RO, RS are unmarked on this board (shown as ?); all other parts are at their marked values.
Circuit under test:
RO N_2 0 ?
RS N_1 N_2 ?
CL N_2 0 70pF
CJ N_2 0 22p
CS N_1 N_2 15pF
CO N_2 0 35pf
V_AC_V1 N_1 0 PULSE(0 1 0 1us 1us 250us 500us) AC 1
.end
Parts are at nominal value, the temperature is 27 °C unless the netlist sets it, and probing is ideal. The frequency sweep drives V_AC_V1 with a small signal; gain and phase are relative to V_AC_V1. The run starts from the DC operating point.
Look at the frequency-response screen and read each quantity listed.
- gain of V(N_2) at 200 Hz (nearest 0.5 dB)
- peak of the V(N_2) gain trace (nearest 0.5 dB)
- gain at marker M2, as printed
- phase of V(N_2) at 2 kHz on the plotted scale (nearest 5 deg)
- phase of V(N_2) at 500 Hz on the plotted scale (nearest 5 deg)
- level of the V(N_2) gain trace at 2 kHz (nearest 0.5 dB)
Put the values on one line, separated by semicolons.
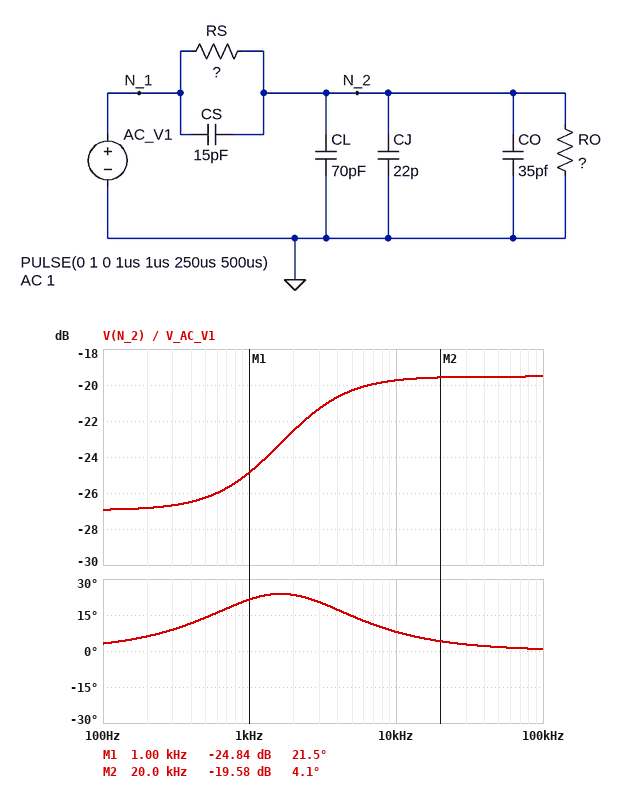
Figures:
-27.0 dB; -19.5 dB; -19.58 dB; 25 deg; 15 deg; -22.5 dB
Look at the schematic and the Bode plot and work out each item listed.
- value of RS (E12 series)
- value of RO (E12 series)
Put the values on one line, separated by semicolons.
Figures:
10 MΩ; 470 kΩ
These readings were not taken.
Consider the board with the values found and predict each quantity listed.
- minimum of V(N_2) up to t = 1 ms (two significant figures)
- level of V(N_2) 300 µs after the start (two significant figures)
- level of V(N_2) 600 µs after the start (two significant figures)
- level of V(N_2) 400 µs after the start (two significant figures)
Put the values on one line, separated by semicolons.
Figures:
-59 mV; -28 mV; 57 mV; -5.8 mV
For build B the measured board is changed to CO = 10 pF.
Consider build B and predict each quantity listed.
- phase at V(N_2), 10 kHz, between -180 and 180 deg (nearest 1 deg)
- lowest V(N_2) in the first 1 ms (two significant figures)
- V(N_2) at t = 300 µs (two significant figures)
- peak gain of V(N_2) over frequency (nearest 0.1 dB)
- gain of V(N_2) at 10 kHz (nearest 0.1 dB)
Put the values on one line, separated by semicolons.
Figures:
11 deg; -82 mV; -33 mV; -17.8 dB; -18.2 dB
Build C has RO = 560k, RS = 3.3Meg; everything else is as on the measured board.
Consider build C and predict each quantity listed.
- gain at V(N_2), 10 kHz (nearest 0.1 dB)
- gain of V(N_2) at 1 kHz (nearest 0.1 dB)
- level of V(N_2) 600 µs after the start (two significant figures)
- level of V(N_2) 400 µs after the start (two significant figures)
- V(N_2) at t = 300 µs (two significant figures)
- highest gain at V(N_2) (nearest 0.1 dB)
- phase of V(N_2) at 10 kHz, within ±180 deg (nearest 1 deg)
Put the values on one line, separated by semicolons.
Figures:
-19.3 dB; -17.1 dB; 140 mV; 4.3 mV; 19 mV; -16.8 dB; -5 deg
